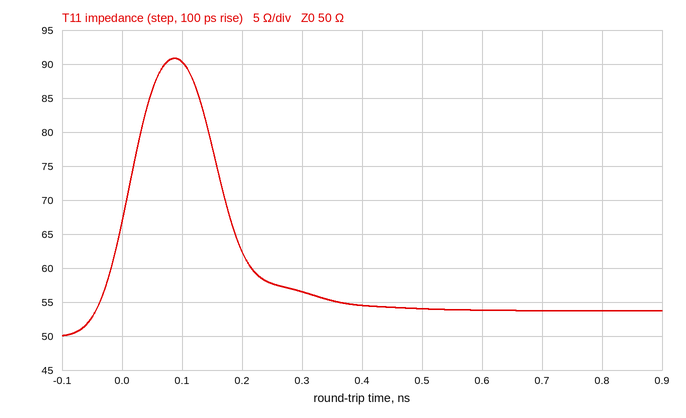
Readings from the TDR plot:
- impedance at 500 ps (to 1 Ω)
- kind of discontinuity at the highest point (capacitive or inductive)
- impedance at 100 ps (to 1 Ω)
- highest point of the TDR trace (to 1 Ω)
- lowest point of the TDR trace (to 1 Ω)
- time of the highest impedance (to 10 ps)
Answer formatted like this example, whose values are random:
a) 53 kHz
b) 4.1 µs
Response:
a) 54 Ω
b) inductive
c) 90 Ω
d) 91 Ω
e) 50 Ω
f) 90 ps
